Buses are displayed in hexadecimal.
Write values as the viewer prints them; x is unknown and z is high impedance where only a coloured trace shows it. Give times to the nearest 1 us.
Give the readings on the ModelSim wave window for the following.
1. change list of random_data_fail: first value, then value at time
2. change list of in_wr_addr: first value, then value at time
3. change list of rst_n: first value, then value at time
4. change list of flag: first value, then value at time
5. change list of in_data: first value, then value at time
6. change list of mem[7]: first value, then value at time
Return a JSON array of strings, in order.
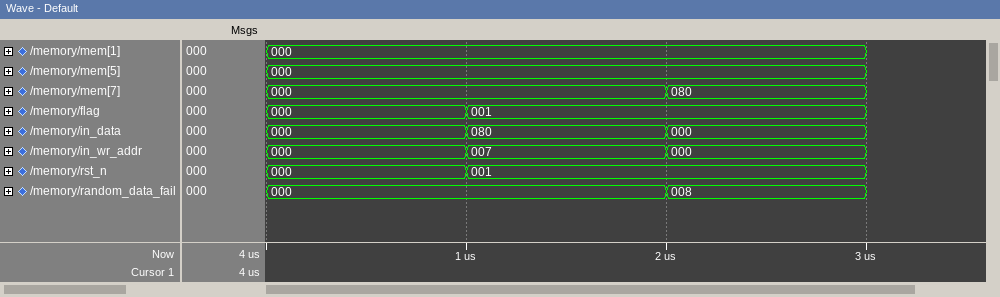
["000, 008 at 2 us", "000, 007 at 1 us, 000 at 2 us", "000, 001 at 1 us", "000, 001 at 1 us", "000, 080 at 1 us, 000 at 2 us", "000, 080 at 2 us"]
